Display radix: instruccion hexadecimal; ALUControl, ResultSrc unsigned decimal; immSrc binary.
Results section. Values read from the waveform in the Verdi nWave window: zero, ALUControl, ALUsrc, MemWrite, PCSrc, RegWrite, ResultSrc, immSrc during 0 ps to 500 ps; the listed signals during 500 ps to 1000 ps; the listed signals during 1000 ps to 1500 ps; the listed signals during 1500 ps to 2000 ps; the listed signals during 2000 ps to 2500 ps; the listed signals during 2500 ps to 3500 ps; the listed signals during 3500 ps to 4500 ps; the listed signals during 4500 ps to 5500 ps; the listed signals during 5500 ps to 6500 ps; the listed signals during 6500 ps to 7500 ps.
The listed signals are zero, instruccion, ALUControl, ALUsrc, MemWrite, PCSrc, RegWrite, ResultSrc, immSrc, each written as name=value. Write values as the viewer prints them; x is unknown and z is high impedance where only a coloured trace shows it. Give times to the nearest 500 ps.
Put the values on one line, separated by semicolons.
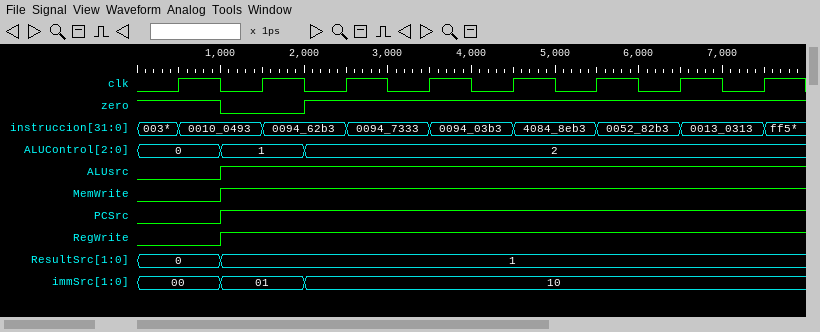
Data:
zero=1, ALUControl=0, ALUsrc=0, MemWrite=0, PCSrc=0, RegWrite=0, ResultSrc=0, immSrc=00; zero=1, instruccion=0010_0493, ALUControl=0, ALUsrc=0, MemWrite=0, PCSrc=0, RegWrite=0, ResultSrc=0, immSrc=00; zero=0, instruccion=0010_0493, ALUControl=1, ALUsrc=1, MemWrite=1, PCSrc=1, RegWrite=1, ResultSrc=1, immSrc=01; zero=0, instruccion=0094_62b3, ALUControl=1, ALUsrc=1, MemWrite=1, PCSrc=1, RegWrite=1, ResultSrc=1, immSrc=01; zero=1, instruccion=0094_62b3, ALUControl=2, ALUsrc=1, MemWrite=1, PCSrc=1, RegWrite=1, ResultSrc=1, immSrc=10; zero=1, instruccion=0094_7333, ALUControl=2, ALUsrc=1, MemWrite=1, PCSrc=1, RegWrite=1, ResultSrc=1, immSrc=10; zero=1, instruccion=0094_03b3, ALUControl=2, ALUsrc=1, MemWrite=1, PCSrc=1, RegWrite=1, ResultSrc=1, immSrc=10; zero=1, instruccion=4084_8eb3, ALUControl=2, ALUsrc=1, MemWrite=1, PCSrc=1, RegWrite=1, ResultSrc=1, immSrc=10; zero=1, instruccion=0052_82b3, ALUControl=2, ALUsrc=1, MemWrite=1, PCSrc=1, RegWrite=1, ResultSrc=1, immSrc=10; zero=1, instruccion=0013_0313, ALUControl=2, ALUsrc=1, MemWrite=1, PCSrc=1, RegWrite=1, ResultSrc=1, immSrc=10
